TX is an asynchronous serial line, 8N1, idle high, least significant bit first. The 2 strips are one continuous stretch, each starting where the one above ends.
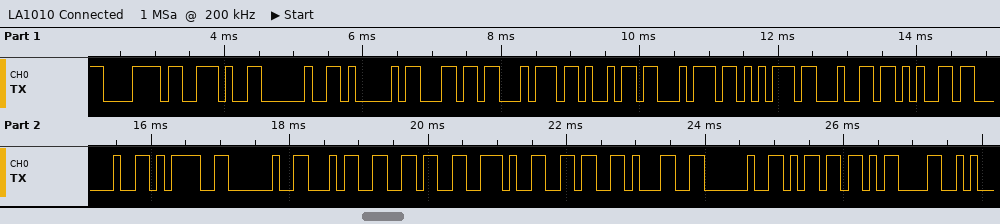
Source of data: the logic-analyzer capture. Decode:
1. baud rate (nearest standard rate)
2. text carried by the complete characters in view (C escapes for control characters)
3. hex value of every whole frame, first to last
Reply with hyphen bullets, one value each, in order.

- 9600 baud
- "x. Altitude = 46.61 m\r"
- 78 2E 20 41 6C 74 69 74 75 64 65 20 3D 20 34 36 2E 36 31 20 6D 0D
